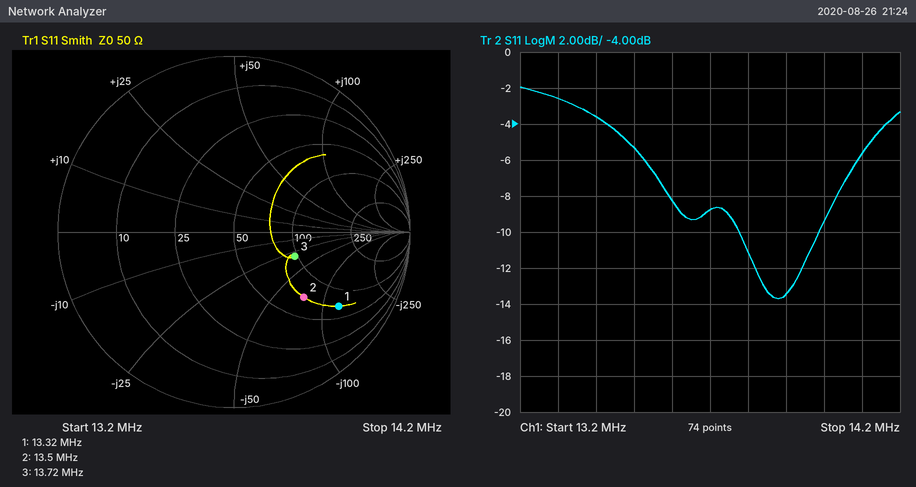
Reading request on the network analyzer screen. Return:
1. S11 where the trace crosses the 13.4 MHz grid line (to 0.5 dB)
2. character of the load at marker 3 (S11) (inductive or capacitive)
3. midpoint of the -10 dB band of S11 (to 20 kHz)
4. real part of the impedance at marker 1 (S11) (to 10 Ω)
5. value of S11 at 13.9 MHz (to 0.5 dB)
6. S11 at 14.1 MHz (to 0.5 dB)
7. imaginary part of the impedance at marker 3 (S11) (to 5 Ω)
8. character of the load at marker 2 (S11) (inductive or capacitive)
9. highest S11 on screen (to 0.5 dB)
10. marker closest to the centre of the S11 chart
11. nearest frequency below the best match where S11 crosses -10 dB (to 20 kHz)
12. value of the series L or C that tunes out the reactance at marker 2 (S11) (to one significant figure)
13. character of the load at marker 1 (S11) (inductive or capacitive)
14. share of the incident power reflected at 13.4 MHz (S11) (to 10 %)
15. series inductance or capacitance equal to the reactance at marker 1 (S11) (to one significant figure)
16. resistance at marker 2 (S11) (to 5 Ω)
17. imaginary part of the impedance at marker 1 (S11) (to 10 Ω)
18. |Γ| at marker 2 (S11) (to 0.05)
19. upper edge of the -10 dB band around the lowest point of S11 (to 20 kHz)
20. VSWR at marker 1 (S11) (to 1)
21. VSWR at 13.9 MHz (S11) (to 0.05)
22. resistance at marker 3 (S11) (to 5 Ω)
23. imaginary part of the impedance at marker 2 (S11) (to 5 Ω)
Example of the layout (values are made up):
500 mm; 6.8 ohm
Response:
-3.5 dB; capacitive; 13.88 MHz; 70 Ω; -13.5 dB; -5.5 dB; -30 Ω; capacitive; -2.0 dB; marker 3; 13.78 MHz; 900 nH; capacitive; 40 %; 100 pF; 70 Ω; -120 Ω; 0.55; 13.98 MHz; 6; 1.55; 95 Ω; -75 Ω
